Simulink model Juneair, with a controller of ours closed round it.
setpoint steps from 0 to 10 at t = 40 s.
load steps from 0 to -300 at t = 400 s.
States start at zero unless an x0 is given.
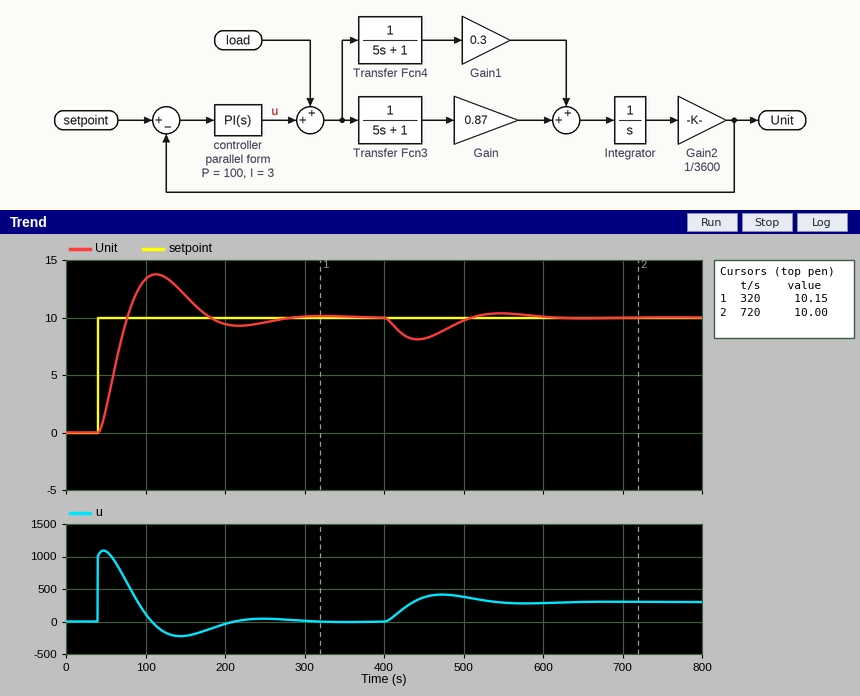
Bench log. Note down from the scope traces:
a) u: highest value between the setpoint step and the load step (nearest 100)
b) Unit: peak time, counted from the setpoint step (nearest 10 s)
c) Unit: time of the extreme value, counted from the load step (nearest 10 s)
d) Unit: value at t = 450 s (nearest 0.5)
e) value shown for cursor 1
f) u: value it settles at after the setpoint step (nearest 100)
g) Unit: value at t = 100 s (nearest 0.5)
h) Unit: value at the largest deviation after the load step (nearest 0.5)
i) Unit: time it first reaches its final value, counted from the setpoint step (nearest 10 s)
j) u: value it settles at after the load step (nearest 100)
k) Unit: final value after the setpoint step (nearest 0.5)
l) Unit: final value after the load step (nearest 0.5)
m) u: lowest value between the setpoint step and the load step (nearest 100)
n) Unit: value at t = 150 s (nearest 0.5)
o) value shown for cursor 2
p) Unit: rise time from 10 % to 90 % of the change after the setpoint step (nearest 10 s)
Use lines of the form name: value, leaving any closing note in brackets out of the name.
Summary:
u: highest value between the setpoint step and the load step: 1100
Unit: peak time, counted from the setpoint step: 70 s
Unit: time of the extreme value, counted from the load step: 40 s
Unit: value at t = 450 s: 8.0
value shown for cursor 1: 10.15
u: value it settles at after the setpoint step: 0
Unit: value at t = 100 s: 13.5
Unit: value at the largest deviation after the load step: 8.0
Unit: time it first reaches its final value, counted from the setpoint step: 40 s
u: value it settles at after the load step: 300
Unit: final value after the setpoint step: 10.0
Unit: final value after the load step: 10.0
u: lowest value between the setpoint step and the load step: -200
Unit: value at t = 150 s: 12.0
value shown for cursor 2: 10.00
Unit: rise time from 10 % to 90 % of the change after the setpoint step: 30 s
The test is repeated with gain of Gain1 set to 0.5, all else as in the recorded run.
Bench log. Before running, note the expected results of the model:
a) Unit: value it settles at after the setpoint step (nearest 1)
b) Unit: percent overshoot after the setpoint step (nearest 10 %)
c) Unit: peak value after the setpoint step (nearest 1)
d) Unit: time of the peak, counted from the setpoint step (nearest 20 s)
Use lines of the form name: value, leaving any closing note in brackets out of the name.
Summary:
Unit: value it settles at after the setpoint step: 10
Unit: percent overshoot after the setpoint step: 40 %
Unit: peak value after the setpoint step: 14
Unit: time of the peak, counted from the setpoint step: 60 s
